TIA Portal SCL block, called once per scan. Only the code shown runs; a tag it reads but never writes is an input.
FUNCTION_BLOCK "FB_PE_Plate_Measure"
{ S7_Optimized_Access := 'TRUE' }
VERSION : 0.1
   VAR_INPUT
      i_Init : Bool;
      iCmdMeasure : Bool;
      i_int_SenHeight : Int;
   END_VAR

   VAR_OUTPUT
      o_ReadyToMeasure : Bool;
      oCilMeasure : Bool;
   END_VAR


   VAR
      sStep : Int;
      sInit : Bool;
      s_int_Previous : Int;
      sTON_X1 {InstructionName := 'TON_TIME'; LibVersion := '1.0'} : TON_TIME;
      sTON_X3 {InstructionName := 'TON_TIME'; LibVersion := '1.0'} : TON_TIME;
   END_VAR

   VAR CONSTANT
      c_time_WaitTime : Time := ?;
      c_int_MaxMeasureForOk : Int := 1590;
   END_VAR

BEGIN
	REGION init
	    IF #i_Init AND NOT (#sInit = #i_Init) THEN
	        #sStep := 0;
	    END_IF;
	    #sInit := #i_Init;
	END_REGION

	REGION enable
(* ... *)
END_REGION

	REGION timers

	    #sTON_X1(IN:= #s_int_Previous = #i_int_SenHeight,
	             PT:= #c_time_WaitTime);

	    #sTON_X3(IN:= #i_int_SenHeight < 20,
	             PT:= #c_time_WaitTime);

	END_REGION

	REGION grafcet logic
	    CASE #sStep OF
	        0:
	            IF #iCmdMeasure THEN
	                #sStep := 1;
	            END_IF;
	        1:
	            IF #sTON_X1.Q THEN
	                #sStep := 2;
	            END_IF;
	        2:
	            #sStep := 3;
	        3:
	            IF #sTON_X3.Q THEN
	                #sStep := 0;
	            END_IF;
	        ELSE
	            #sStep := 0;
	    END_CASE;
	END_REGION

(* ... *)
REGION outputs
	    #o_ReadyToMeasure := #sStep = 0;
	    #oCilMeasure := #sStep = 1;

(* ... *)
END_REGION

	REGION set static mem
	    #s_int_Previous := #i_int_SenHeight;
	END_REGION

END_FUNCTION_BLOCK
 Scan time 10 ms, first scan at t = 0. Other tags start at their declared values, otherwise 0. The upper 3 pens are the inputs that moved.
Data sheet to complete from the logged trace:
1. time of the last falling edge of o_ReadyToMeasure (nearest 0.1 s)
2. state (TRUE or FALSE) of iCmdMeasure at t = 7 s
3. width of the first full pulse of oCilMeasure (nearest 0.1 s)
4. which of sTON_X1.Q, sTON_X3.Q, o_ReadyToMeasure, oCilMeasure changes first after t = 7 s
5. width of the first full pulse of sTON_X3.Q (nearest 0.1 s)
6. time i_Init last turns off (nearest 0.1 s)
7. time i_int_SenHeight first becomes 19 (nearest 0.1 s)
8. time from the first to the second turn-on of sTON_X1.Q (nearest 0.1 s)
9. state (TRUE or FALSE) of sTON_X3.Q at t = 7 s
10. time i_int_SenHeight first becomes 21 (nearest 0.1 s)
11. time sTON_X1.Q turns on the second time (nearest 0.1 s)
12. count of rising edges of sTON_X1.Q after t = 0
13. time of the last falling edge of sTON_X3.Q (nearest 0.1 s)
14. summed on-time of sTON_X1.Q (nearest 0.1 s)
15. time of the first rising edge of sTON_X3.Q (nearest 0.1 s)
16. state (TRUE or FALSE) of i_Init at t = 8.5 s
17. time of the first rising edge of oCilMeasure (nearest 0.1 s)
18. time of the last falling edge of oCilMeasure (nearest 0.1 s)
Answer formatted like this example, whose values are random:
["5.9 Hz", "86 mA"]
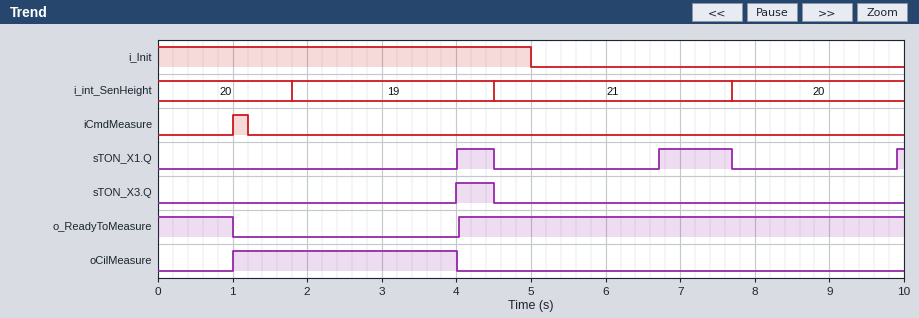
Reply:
["1.0 s", "FALSE", "3.0 s", "sTON_X1.Q", "0.5 s", "5.0 s", "1.8 s", "2.7 s", "FALSE", "4.5 s", "6.7 s", "3", "4.5 s", "1.6 s", "4.0 s", "FALSE", "1.0 s", "4.0 s"]
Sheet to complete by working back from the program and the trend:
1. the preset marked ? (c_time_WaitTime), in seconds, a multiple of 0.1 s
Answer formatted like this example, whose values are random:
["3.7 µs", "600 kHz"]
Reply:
["2.2 s"]
